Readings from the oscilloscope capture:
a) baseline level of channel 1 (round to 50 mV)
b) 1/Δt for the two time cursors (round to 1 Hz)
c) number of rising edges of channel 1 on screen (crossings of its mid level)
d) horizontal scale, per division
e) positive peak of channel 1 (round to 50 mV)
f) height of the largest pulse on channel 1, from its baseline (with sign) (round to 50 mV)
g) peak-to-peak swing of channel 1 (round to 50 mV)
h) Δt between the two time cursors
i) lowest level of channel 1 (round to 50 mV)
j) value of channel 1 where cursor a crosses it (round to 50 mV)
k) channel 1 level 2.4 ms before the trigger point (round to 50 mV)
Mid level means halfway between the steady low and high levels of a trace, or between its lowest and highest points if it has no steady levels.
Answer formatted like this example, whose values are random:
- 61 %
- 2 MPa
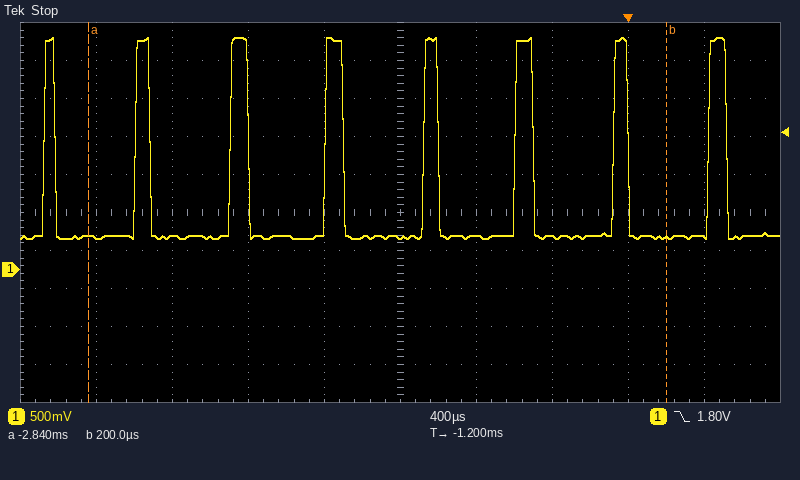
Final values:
- 450 mV
- 329 Hz
- 8
- 400 µs
- 3.05 V
- +2.60 V
- 2.65 V
- 3.04 ms
- 400 mV
- 450 mV
- 450 mV
